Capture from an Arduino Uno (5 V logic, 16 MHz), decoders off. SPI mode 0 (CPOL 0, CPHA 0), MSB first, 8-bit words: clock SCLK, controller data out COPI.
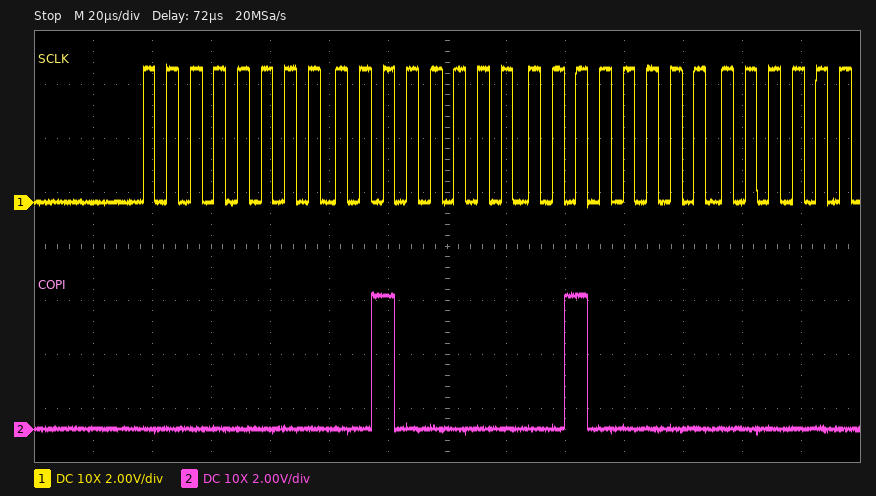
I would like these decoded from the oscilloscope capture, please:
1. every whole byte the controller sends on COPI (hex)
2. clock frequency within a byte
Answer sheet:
00 20 20
125 kHz
